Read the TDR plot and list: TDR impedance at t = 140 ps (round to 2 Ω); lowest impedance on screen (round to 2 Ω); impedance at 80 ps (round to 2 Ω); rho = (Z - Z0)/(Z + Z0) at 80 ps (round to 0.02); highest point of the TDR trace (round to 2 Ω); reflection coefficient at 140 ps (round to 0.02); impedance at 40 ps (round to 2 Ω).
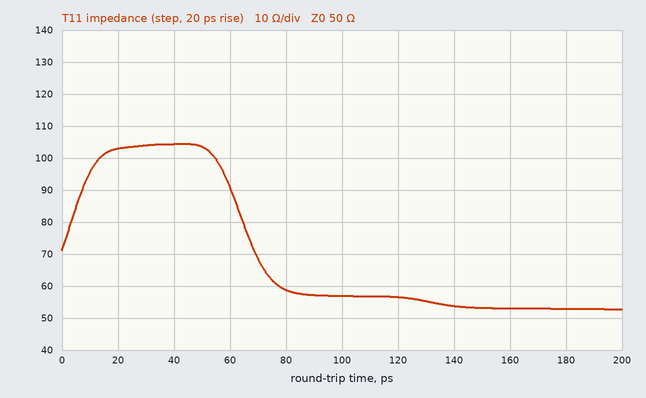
54 Ω
52 Ω
58 Ω
+0.08
104 Ω
+0.04
104 Ω
